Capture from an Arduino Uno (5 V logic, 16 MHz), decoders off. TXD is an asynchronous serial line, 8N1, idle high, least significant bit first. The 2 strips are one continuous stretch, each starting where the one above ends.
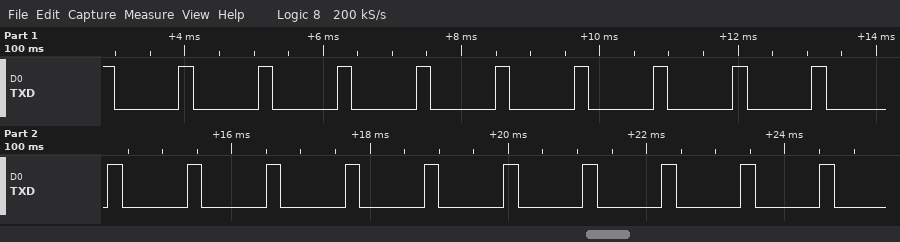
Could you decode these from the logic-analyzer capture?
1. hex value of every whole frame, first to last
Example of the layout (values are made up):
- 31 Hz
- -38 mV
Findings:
- 00 00 00 00 00 00 00 00 00 00 00 00 00 00 00 00 00 00 00
